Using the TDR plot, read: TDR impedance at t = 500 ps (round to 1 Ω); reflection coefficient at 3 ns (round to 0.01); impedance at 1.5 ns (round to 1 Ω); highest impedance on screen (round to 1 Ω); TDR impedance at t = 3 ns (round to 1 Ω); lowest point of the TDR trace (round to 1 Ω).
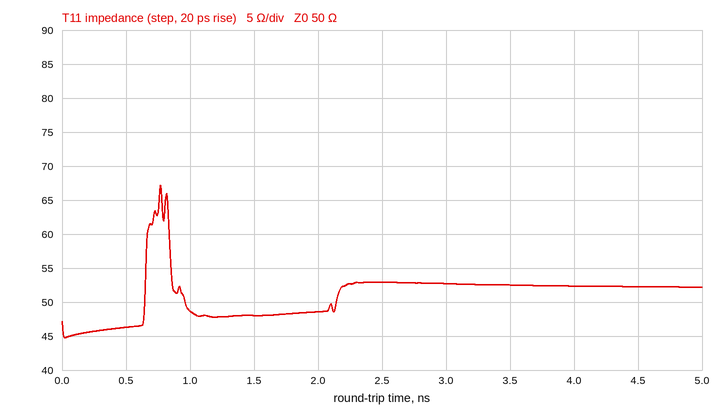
46 Ω
+0.03
48 Ω
67 Ω
53 Ω
45 Ω
